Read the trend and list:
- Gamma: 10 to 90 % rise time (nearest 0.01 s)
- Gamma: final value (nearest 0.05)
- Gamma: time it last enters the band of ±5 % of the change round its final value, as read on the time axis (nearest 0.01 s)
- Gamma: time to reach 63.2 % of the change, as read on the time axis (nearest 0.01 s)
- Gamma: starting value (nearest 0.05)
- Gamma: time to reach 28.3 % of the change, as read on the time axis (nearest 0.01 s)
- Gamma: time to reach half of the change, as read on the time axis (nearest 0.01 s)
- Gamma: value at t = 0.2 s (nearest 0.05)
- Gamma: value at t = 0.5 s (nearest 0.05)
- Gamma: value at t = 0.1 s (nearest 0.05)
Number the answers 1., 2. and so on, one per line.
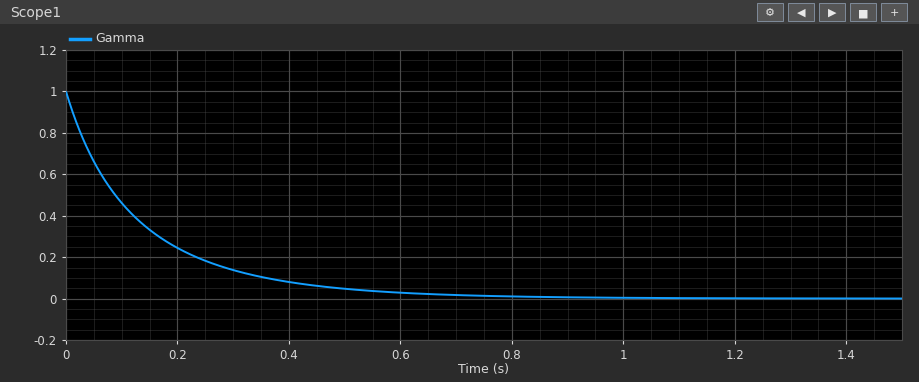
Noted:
1. 0.35 s
2. 0.00
3. 0.49 s
4. 0.13 s
5. 1.00
6. 0.04 s
7. 0.09 s
8. 0.25
9. 0.05
10. 0.45
